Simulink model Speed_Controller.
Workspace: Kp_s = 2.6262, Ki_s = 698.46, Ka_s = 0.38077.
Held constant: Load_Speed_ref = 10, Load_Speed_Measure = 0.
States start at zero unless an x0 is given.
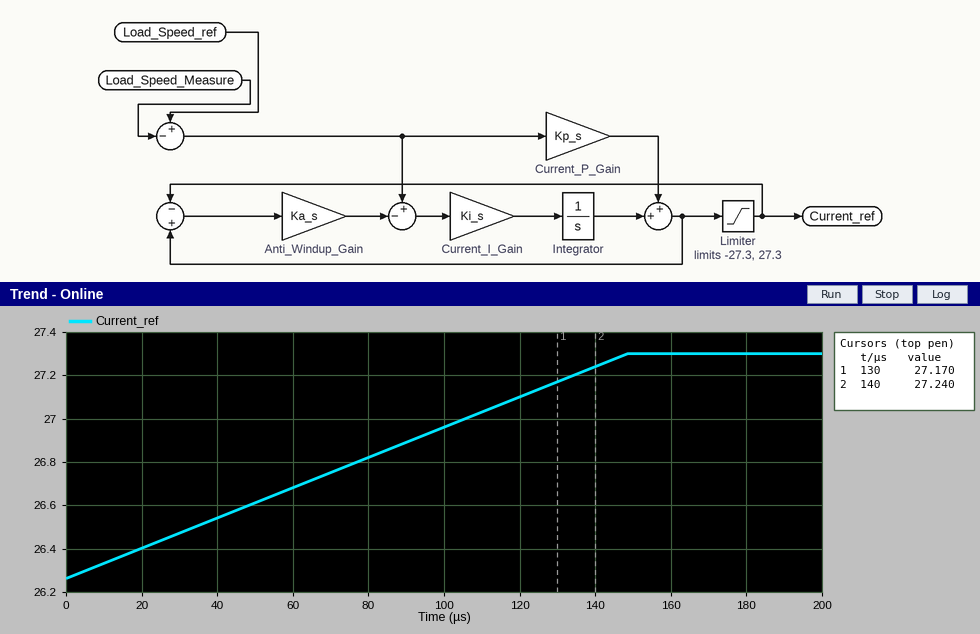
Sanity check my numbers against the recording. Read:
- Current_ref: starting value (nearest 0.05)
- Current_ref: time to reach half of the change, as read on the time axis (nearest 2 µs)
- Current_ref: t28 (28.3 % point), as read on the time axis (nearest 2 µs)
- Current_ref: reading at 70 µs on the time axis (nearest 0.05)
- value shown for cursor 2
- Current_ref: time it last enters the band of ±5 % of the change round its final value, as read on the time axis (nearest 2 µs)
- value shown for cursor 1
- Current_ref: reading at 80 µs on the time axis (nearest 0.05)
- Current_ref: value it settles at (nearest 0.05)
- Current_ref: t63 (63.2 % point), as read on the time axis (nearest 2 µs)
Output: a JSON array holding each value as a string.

["26.25", "74 µs", "42 µs", "26.75", "27.240", "142 µs", "27.170", "26.80", "27.30", "94 µs"]
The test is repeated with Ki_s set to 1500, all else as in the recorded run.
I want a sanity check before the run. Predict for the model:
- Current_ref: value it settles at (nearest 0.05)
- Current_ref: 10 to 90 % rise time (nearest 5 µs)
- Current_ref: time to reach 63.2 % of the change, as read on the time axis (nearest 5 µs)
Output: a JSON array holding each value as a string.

["27.30", "55 µs", "45 µs"]
